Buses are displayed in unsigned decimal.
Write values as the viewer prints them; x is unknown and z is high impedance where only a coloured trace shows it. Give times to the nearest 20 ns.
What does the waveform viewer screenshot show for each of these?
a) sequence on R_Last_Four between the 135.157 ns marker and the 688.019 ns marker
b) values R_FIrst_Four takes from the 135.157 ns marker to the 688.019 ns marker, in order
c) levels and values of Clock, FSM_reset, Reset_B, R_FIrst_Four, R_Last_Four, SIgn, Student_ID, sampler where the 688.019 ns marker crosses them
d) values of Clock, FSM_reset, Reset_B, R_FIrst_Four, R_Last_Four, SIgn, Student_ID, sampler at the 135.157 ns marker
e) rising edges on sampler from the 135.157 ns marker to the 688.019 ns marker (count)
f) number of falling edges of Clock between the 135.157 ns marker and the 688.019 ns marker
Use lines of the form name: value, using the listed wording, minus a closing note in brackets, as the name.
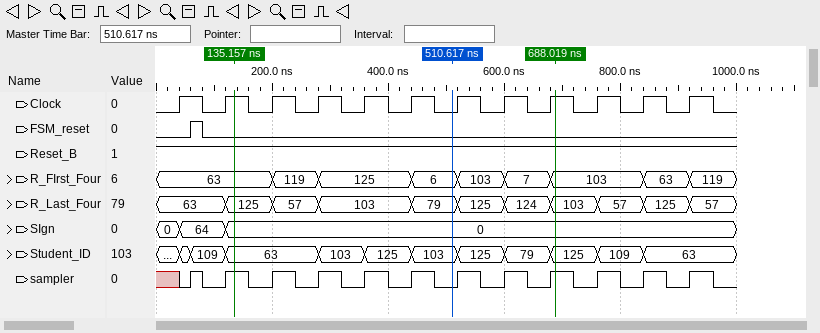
sequence on R_Last_Four between the 135.157 ns marker and the 688.019 ns marker: 125, 57, 103, 79, 125, 124, 103
values R_FIrst_Four takes from the 135.157 ns marker to the 688.019 ns marker, in order: 63, 119, 125, 6, 103, 7, 103
levels and values of Clock, FSM_reset, Reset_B, R_FIrst_Four, R_Last_Four, SIgn, Student_ID, sampler where the 688.019 ns marker crosses them: Clock=1, FSM_reset=0, Reset_B=1, R_FIrst_Four=103, R_Last_Four=103, SIgn=0, Student_ID=125, sampler=1
values of Clock, FSM_reset, Reset_B, R_FIrst_Four, R_Last_Four, SIgn, Student_ID, sampler at the 135.157 ns marker: Clock=1, FSM_reset=0, Reset_B=1, R_FIrst_Four=63, R_Last_Four=125, SIgn=0, Student_ID=63, sampler=1
rising edges on sampler from the 135.157 ns marker to the 688.019 ns marker: 7
number of falling edges of Clock between the 135.157 ns marker and the 688.019 ns marker: 7
